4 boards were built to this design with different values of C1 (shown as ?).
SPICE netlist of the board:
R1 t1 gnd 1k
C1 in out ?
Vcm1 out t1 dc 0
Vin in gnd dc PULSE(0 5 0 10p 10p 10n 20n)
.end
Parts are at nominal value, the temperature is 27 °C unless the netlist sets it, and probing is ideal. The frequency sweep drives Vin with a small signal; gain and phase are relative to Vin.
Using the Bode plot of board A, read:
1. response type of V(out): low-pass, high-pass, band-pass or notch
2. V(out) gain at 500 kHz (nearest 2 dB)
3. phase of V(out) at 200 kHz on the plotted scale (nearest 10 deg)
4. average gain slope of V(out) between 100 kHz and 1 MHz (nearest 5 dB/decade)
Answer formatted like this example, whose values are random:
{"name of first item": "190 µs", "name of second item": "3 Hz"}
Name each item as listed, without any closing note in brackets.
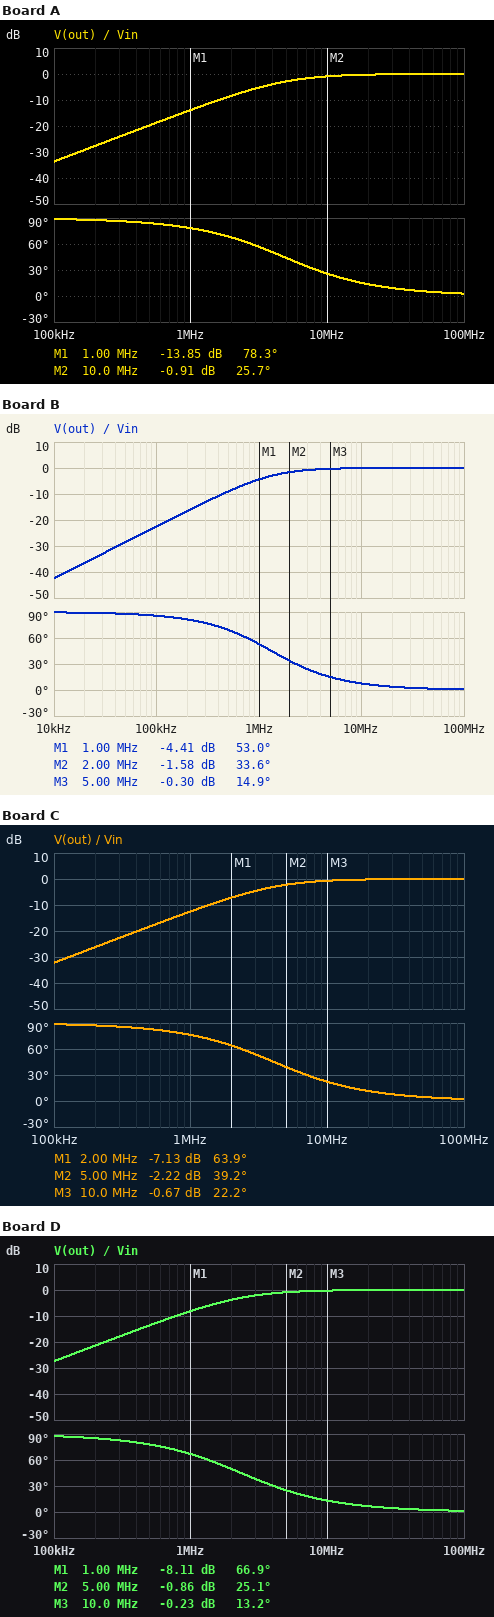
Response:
{"response type of V(out): low-pass, high-pass, band-pass or notch": "high-pass", "V(out) gain at 500 kHz": "-20 dB", "phase of V(out) at 200 kHz on the plotted scale": "90 deg", "average gain slope of V(out) between 100 kHz and 1 MHz": "20 dB/decade"}
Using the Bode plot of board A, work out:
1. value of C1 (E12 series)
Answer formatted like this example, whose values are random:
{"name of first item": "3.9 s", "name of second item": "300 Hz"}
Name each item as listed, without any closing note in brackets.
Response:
{"value of C1": "33 pF"}
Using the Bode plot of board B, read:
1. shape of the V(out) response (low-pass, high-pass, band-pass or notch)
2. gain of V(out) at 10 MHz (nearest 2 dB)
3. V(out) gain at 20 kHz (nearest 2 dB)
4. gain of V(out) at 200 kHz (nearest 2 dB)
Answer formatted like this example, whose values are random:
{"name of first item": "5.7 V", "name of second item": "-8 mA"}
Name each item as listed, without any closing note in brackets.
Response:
{"shape of the V(out) response": "high-pass", "gain of V(out) at 10 MHz": "0 dB", "V(out) gain at 20 kHz": "-36 dB", "gain of V(out) at 200 kHz": "-16 dB"}
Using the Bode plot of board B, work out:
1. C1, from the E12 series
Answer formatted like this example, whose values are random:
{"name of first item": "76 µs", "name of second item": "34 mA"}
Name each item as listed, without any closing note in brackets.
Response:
{"C1, from the E12 series": "120 pF"}
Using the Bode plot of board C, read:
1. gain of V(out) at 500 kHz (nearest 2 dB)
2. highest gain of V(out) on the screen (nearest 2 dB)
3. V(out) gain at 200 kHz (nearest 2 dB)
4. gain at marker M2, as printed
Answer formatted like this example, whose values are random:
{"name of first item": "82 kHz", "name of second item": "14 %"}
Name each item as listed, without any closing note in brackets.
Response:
{"gain of V(out) at 500 kHz": "-18 dB", "highest gain of V(out) on the screen": "0 dB", "V(out) gain at 200 kHz": "-26 dB", "gain at marker M2, as printed": "-2.22 dB"}
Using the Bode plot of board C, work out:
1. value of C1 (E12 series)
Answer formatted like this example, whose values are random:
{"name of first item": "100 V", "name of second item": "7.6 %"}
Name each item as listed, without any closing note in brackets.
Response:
{"value of C1": "39 pF"}
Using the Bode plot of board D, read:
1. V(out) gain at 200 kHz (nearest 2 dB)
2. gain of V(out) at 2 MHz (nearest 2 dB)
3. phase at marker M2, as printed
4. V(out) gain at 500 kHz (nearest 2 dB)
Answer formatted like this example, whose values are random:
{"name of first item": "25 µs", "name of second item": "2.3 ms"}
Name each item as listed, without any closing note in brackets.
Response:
{"V(out) gain at 200 kHz": "-22 dB", "gain of V(out) at 2 MHz": "-4 dB", "phase at marker M2, as printed": "25.1 deg", "V(out) gain at 500 kHz": "-14 dB"}
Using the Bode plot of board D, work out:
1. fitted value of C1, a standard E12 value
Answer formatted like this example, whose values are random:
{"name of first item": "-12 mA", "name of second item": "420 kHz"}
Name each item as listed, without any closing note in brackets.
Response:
{"fitted value of C1, a standard E12 value": "68 pF"}
